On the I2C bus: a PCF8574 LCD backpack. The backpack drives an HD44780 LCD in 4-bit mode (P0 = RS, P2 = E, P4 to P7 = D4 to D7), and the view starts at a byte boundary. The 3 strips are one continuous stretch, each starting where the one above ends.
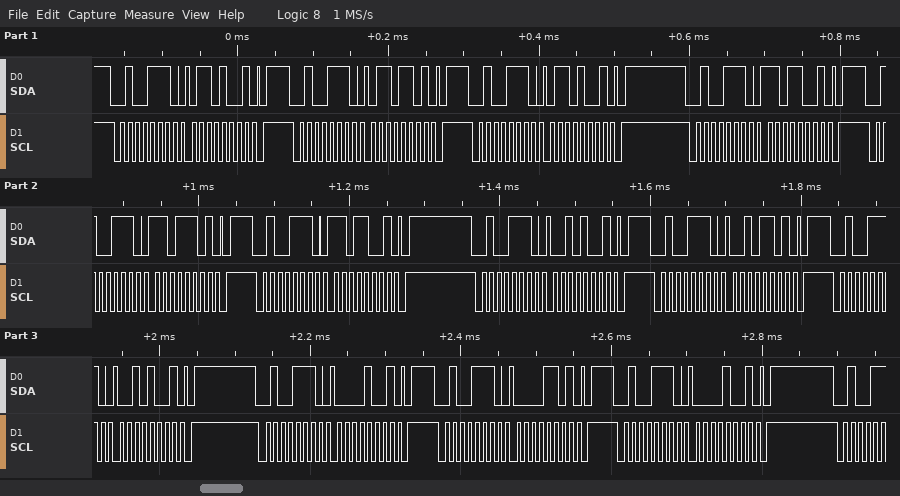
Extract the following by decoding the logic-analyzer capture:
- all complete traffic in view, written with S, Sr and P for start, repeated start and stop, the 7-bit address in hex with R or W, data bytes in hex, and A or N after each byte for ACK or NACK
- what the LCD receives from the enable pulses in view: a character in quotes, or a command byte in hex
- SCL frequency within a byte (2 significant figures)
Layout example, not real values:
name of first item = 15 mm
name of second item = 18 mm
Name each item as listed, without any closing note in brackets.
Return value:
all complete traffic in view, written with S, Sr and P for start, repeated start and stop, the 7-bit address in hex with R or W, data bytes in hex, and A or N after each byte for ACK or NACK = S 27W A 69 A P S 27W A 6D A P S 27W A 69 A P S 27W A D9 A P S 27W A DD A P S 27W A D9 A P S 27W A 29 A P S 27W A 2D A P S 27W A 29 A P S 27W A 09 A P S 27W A 0D A P S 27W A 09 A P
what the LCD receives from the enable pulses in view: a character in quotes, or a command byte in hex = 'm' ' '
SCL frequency within a byte = 100 kHz
